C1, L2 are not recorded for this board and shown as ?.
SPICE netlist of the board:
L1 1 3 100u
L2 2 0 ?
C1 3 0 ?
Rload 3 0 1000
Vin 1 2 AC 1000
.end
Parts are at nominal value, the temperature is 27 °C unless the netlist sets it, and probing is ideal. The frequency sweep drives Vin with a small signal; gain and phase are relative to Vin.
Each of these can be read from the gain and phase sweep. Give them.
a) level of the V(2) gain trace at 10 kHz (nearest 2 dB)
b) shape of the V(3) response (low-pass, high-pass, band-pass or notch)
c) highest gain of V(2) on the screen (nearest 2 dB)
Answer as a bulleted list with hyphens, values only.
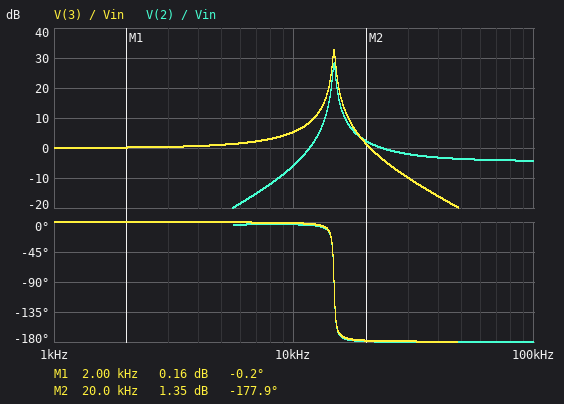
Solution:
- -6 dB
- low-pass
- 28 dB
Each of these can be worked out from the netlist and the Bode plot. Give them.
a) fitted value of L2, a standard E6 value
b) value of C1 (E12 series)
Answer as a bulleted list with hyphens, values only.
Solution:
- 150 µH
- 470 nF
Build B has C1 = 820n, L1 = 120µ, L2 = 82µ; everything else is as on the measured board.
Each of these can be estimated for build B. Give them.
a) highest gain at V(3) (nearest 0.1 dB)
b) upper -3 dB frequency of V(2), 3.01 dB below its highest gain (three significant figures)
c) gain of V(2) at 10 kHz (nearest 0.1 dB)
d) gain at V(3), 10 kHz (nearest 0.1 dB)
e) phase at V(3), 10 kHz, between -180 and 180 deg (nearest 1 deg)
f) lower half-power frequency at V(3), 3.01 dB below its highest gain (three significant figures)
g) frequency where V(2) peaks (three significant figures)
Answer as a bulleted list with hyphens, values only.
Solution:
- 36.1 dB
- 12.5 kHz
- -2.3 dB
- 9.2 dB
- -2 deg
- 12.3 kHz
- 12.4 kHz
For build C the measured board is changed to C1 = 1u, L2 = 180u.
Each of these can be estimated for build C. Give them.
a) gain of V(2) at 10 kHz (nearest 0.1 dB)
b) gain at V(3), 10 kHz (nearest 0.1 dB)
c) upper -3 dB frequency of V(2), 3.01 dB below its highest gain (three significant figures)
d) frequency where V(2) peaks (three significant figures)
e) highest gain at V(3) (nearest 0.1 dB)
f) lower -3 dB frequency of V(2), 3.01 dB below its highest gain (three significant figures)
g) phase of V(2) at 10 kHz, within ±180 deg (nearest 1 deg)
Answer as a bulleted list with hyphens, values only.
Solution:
- 16.5 dB
- 19.4 dB
- 9.59 kHz
- 9.51 kHz
- 35.5 dB
- 9.43 kHz
- -171 deg
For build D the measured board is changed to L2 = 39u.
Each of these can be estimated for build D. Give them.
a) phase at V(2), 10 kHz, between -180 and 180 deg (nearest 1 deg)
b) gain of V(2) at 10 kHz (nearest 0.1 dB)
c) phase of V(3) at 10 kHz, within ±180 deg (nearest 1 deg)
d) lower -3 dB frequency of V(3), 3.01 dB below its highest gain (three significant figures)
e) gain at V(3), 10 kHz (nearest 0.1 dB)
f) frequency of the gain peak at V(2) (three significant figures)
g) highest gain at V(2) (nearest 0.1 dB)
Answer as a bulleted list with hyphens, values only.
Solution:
- -3 deg
- -20.2 dB
- -1 deg
- 19.5 kHz
- 2.6 dB
- 19.7 kHz
- 24.2 dB
